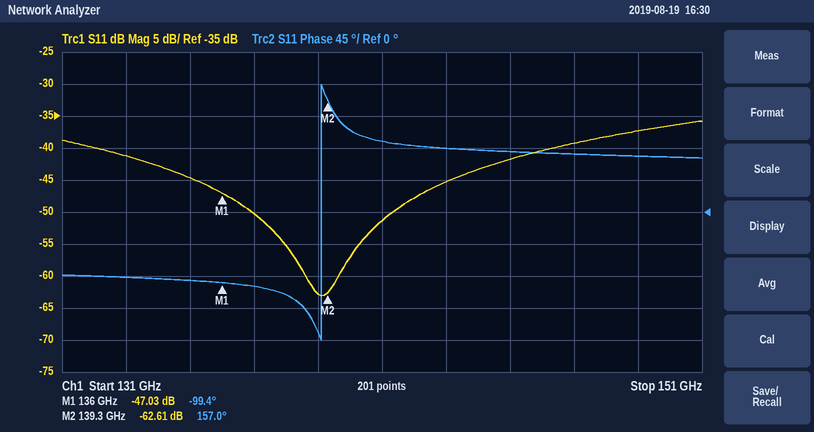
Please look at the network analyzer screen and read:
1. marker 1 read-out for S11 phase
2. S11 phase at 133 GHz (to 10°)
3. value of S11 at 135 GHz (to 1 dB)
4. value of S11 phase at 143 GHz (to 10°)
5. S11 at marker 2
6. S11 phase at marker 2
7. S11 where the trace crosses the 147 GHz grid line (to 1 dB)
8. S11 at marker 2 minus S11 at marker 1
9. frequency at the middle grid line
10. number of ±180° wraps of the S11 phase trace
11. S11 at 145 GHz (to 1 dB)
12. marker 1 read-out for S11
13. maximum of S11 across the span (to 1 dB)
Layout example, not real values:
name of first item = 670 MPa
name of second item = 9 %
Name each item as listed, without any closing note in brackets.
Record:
marker 1 read-out for S11 phase = -99.4°
S11 phase at 133 GHz = -90°
value of S11 at 135 GHz = -45 dB
value of S11 phase at 143 GHz = 90°
S11 at marker 2 = -62.61 dB
S11 phase at marker 2 = 157.0°
S11 where the trace crosses the 147 GHz grid line = -39 dB
S11 at marker 2 minus S11 at marker 1 = -15.58 dB
frequency at the middle grid line = 141 GHz
number of ±180° wraps of the S11 phase trace = 1
S11 at 145 GHz = -42 dB
marker 1 read-out for S11 = -47.03 dB
maximum of S11 across the span = -36 dB
